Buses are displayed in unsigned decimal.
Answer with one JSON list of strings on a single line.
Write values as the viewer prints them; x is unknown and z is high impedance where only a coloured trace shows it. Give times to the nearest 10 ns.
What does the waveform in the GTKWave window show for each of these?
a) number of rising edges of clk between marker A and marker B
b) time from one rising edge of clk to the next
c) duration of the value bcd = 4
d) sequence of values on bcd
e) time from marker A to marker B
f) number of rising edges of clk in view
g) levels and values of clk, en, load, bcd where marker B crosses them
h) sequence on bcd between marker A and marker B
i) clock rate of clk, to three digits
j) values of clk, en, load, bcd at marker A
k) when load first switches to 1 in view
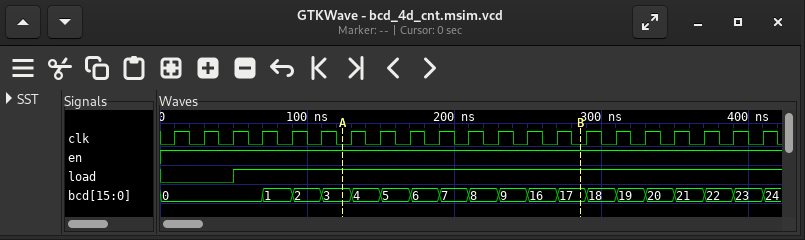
["8", "20 ns", "20 ns", "0, 1, 2, 3, 4, 5, 6, 7, 8, 9, 16, 17, 18, 19, 20, 21, 22, 23, 24", "160 ns", "21", "clk=0, en=1, load=1, bcd=17", "3, 4, 5, 6, 7, 8, 9, 16, 17", "50.0 MHz", "clk=0, en=1, load=1, bcd=3", "50 ns"]
